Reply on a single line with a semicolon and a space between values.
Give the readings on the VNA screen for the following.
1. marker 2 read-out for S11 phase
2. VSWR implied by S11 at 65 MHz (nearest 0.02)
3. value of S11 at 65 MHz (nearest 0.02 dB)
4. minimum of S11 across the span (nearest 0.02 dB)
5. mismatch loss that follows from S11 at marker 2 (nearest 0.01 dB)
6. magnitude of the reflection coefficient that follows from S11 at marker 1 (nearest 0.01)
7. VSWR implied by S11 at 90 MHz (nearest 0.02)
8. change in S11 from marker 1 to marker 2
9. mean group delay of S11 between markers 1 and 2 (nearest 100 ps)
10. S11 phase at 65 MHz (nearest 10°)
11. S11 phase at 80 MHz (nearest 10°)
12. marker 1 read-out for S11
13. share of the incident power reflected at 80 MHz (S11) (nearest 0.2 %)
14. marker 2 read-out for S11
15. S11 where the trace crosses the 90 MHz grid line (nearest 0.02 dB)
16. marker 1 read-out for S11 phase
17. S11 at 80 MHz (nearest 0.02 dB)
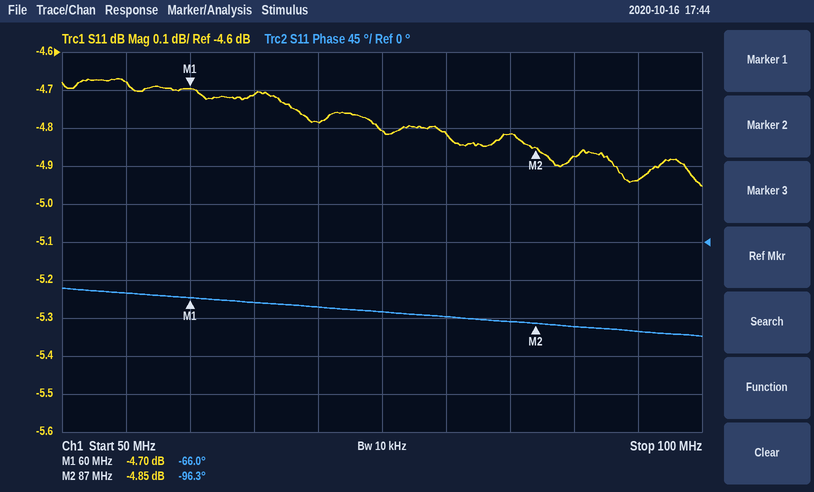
-96.3°; 3.78; -4.72 dB; -4.96 dB; 1.72 dB; 0.58; 3.66; -0.15 dB; 3.1 ns; -70°; -90°; -4.70 dB; 33.0 %; -4.85 dB; -4.88 dB; -66.0°; -4.82 dB
